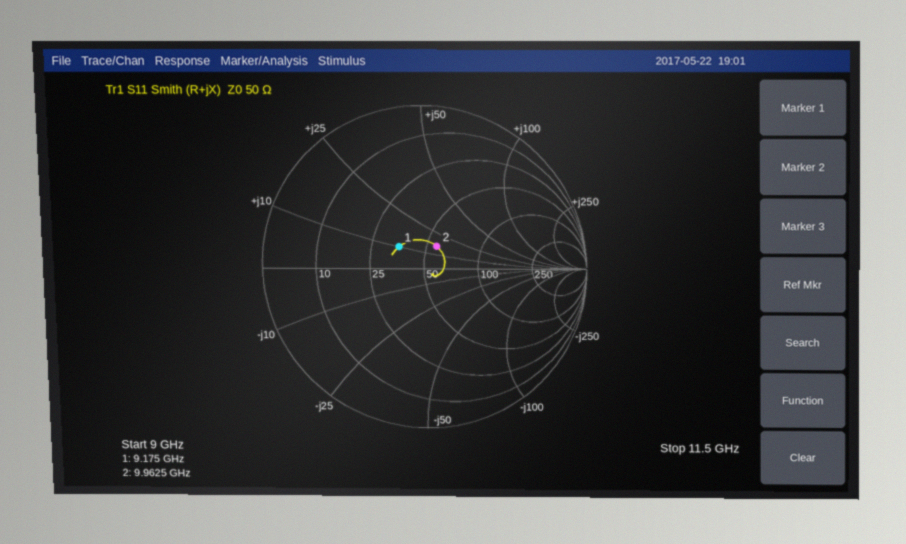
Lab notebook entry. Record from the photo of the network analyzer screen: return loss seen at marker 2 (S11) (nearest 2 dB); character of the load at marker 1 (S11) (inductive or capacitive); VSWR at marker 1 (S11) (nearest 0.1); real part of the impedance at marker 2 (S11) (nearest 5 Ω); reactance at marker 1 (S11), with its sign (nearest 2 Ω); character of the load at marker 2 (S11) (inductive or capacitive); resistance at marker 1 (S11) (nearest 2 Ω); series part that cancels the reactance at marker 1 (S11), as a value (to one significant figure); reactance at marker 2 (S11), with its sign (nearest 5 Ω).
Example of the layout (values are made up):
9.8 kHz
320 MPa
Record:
16 dB
inductive
1.5
55 Ω
+10 Ω
inductive
36 Ω
2 pF
+15 Ω
